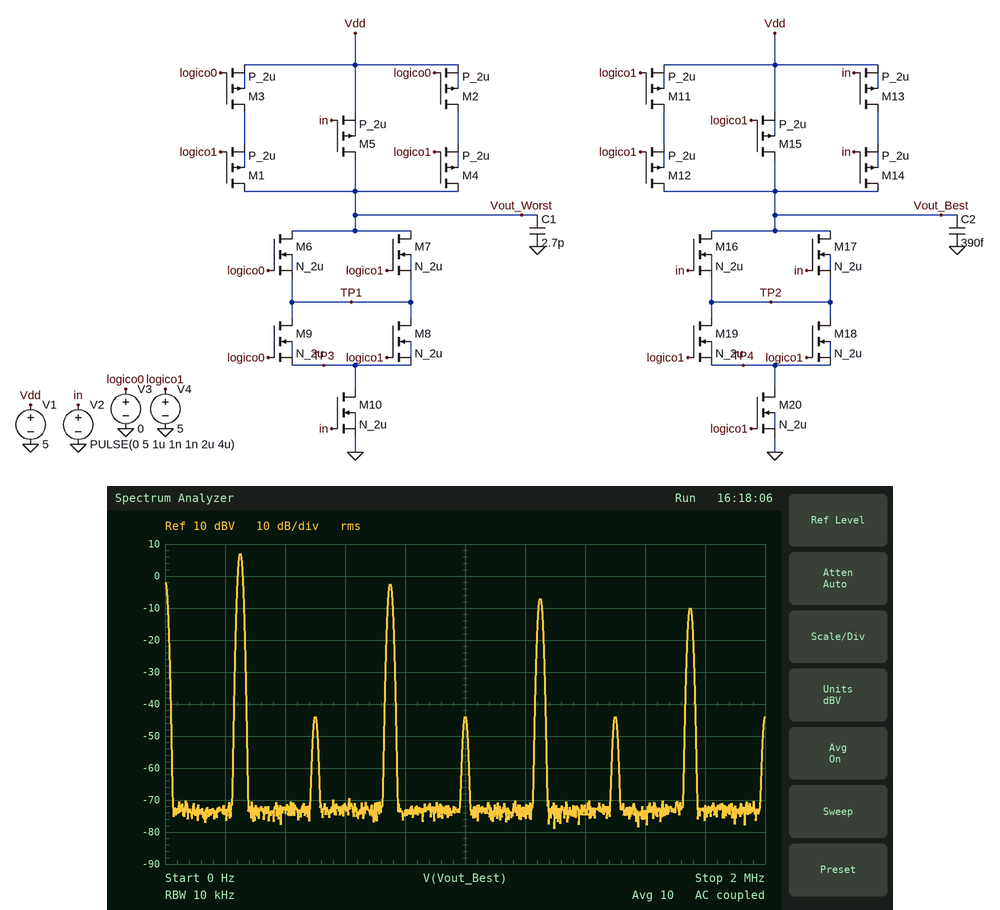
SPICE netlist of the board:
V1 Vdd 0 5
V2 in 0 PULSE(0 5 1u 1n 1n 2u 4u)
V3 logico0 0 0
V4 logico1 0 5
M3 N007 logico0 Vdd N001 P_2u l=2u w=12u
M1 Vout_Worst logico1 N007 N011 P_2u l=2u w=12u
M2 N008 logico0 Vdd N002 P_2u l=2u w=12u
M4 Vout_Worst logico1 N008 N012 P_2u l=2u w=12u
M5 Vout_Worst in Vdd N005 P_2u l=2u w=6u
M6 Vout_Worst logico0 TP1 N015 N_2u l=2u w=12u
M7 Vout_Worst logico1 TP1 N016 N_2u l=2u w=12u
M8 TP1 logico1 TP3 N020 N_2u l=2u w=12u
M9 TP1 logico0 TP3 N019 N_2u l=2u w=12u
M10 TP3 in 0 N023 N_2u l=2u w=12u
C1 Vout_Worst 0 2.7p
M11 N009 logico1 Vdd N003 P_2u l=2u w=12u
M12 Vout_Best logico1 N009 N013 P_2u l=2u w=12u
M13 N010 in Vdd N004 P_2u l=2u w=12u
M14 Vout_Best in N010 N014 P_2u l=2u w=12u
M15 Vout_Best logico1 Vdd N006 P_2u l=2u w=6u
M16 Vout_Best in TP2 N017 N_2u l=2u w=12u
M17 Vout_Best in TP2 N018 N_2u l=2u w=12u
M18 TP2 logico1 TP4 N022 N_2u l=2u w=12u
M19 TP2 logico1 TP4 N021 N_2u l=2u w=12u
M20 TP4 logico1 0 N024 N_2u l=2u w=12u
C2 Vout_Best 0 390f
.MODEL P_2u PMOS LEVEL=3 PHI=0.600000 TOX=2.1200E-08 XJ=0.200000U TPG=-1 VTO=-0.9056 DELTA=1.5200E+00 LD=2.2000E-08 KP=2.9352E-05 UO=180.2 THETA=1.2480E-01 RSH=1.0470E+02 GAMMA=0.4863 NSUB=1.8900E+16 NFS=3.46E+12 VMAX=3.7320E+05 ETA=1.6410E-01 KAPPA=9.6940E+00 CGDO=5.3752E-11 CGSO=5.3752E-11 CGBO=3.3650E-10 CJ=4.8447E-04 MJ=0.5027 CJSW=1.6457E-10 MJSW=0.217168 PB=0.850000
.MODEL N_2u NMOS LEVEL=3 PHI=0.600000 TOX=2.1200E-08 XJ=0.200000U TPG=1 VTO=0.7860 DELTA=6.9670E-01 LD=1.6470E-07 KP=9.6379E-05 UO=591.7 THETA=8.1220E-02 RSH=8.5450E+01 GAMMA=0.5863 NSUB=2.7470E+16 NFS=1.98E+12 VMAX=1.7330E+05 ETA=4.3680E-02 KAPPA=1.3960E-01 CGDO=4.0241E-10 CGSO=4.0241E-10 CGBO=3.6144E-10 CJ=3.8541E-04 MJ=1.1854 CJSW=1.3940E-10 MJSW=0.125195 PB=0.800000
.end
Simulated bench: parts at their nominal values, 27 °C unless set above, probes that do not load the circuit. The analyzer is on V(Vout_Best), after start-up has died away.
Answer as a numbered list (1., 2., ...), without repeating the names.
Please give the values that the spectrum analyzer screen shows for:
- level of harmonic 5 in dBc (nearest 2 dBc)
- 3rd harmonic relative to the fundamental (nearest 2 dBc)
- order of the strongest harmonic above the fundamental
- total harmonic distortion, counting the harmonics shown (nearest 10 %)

1. -14 dBc
2. -10 dBc
3. 3
4. 40 %
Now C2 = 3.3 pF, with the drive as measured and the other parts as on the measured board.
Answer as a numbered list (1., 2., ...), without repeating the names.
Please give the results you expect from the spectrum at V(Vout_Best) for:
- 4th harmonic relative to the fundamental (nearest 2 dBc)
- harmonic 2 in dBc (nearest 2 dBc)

1. -36 dBc
2. -36 dBc
